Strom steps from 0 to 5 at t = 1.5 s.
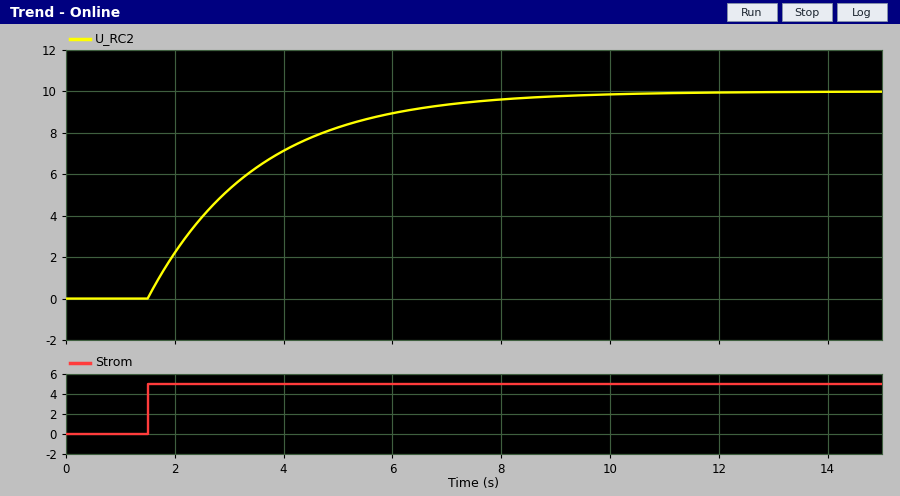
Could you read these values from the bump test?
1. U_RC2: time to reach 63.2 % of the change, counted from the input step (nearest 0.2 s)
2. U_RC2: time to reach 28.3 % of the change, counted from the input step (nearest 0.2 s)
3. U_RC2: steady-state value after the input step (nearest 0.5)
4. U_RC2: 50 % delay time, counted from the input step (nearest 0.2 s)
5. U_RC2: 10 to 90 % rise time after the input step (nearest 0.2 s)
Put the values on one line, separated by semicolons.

2.0 s; 0.6 s; 10.0; 1.4 s; 4.4 s
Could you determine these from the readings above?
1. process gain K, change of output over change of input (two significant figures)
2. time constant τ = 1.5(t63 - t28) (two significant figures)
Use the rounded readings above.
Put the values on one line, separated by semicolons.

2.0; 2.1 s
